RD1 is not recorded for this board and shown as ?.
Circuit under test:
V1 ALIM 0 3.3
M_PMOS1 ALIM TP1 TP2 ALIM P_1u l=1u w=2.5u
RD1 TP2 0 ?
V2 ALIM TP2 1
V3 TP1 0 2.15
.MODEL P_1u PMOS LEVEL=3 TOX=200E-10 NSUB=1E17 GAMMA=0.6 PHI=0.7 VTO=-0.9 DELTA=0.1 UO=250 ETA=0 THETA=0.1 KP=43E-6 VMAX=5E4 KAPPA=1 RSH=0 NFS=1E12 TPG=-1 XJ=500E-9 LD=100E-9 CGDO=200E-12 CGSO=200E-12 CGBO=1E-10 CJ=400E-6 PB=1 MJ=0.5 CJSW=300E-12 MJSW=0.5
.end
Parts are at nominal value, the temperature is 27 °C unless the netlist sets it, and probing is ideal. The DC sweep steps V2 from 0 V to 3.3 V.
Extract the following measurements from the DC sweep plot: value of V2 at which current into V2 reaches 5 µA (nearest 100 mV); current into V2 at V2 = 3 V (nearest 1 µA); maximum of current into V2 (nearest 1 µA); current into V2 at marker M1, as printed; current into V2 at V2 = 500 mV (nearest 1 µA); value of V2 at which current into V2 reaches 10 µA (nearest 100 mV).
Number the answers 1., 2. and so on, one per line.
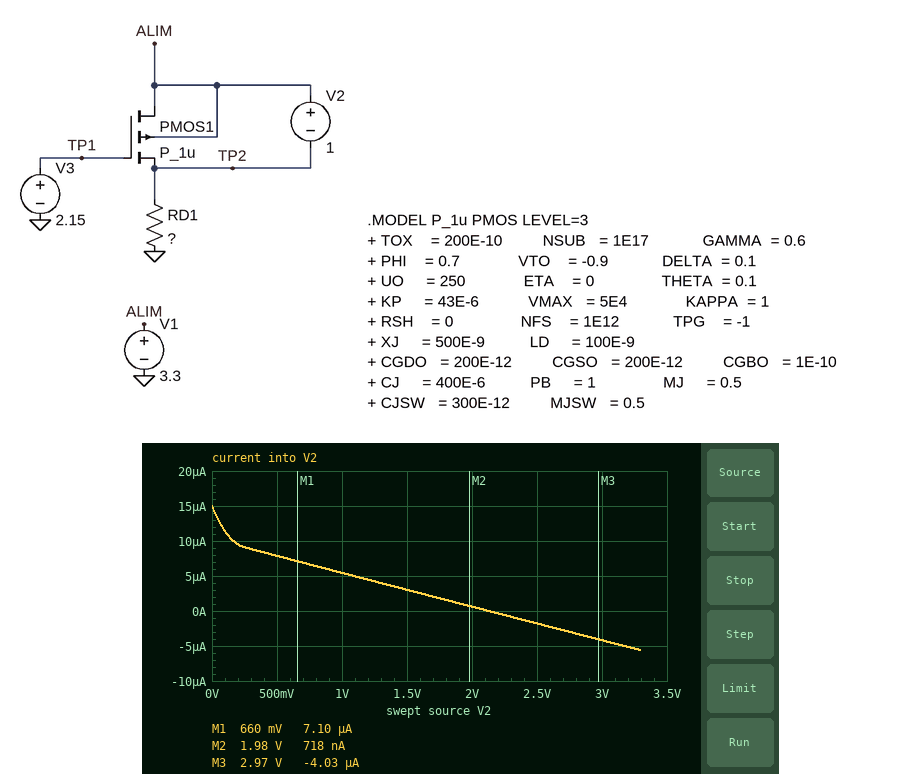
1. 1.1 V
2. -4 µA
3. 15 µA
4. 7.10 µA
5. 8 µA
6. 200 mV
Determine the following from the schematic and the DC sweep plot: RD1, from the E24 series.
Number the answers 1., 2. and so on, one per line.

1. 220 kΩ
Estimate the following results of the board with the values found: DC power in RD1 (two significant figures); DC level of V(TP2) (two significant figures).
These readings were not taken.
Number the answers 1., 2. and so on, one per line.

1. 24 µW
2. 2.3 V
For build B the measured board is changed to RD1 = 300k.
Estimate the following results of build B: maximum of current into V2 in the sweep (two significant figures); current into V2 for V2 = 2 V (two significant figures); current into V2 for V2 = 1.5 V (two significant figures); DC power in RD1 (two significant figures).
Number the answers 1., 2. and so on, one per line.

1. 11 µA
2. -950 nA
3. 850 nA
4. 18 µW
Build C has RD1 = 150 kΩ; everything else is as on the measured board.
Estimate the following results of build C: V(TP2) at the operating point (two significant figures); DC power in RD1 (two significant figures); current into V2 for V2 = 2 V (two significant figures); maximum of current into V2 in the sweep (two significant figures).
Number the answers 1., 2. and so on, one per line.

1. 2.3 V
2. 35 µW
3. 3.4 µA
4. 22 µA
